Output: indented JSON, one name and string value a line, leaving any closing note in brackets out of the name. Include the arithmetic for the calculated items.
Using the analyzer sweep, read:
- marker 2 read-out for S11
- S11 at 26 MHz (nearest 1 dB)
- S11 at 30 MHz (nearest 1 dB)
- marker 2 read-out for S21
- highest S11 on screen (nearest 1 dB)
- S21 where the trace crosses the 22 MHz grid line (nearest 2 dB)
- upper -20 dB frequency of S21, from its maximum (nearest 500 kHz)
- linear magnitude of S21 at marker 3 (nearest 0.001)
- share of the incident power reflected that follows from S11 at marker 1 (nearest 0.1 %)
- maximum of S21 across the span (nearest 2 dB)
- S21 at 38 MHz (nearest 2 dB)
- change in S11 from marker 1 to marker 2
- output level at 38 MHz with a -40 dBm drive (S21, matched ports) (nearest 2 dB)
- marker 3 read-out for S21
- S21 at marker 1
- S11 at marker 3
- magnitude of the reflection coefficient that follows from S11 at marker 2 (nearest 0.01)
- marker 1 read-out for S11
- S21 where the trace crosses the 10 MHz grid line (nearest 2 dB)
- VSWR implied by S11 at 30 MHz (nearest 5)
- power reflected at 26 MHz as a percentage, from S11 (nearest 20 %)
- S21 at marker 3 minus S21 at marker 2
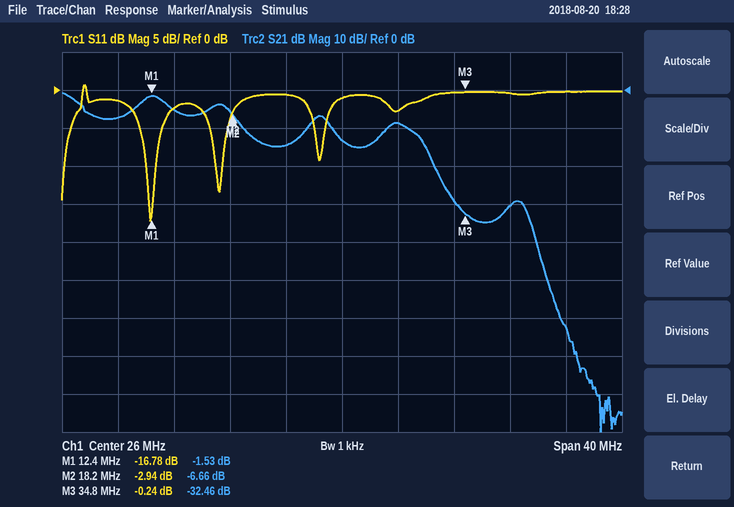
{
  "marker 2 read-out for S11": "-2.94 dB",
  "S11 at 26 MHz": "-1 dB",
  "S11 at 30 MHz": "-3 dB",
  "marker 2 read-out for S21": "-6.66 dB",
  "highest S11 on screen": "1 dB",
  "S21 where the trace crosses the 22 MHz grid line": "-14 dB",
  "upper -20 dB frequency of S21, from its maximum": "32.5 MHz",
  "linear magnitude of S21 at marker 3": "10^(-32.46/20) ≈ 0.024",
  "share of the incident power reflected that follows from S11 at marker 1": "10^(-16.78/10) ≈ 2.1 %",
  "maximum of S21 across the span": "0 dB",
  "S21 at 38 MHz": "-30 dB",
  "change in S11 from marker 1 to marker 2": "-2.94 − (-16.78) = 13.84 dB",
  "output level at 38 MHz with a -40 dBm drive (S21, matched ports)": "-40 dBm + (-30 dB) = -70 dBm",
  "marker 3 read-out for S21": "-32.46 dB",
  "S21 at marker 1": "-1.53 dB",
  "S11 at marker 3": "-0.24 dB",
  "magnitude of the reflection coefficient that follows from S11 at marker 2": "10^(-2.94/20) ≈ 0.71",
  "marker 1 read-out for S11": "-16.78 dB",
  "S21 where the trace crosses the 10 MHz grid line": "-8 dB",
  "VSWR implied by S11 at 30 MHz": "|Γ| = 10^(-3/20) = 0.7079; VSWR = (1 + 0.7079)/(1 − 0.7079) ≈ 5.85, so 5 to the nearest 5",
  "power reflected at 26 MHz as a percentage, from S11": "10^(-1/10) ≈ 79.4 %, so 80 % to the nearest 20 %",
  "S21 at marker 3 minus S21 at marker 2": "-32.46 − (-6.66) = -25.80 dB"
}
